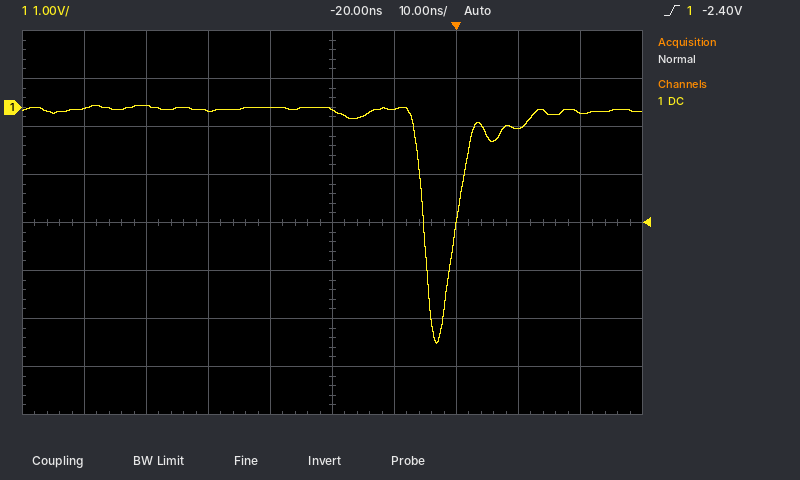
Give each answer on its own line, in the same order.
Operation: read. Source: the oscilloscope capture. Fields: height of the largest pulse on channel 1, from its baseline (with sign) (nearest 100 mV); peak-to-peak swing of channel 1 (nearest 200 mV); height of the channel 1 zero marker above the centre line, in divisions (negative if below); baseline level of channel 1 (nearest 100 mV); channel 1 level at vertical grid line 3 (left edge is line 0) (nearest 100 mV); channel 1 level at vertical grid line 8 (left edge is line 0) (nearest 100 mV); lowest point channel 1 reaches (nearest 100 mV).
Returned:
-4.9 V
5.0 V
+2.4 div
0.0 V
-100 mV
-400 mV
-4.9 V
